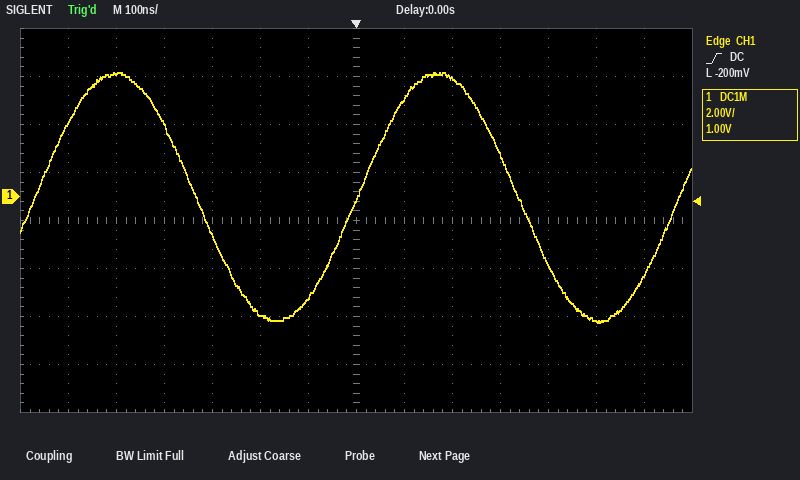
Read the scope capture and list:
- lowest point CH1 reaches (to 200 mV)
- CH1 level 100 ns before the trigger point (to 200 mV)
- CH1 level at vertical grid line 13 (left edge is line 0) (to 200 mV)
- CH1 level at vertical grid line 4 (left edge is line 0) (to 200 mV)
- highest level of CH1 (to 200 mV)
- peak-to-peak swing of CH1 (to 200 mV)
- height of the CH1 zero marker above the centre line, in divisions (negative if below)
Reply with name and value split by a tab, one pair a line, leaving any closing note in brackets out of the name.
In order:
lowest point CH1 reaches	-5.2 V
CH1 level 100 ns before the trigger point	-4.2 V
CH1 level at vertical grid line 13 (left edge is line 0)	-3.2 V
CH1 level at vertical grid line 4 (left edge is line 0)	-1.6 V
highest level of CH1	5.2 V
peak-to-peak swing of CH1	10.4 V
height of the CH1 zero marker above the centre line, in divisions	+0.5 div
